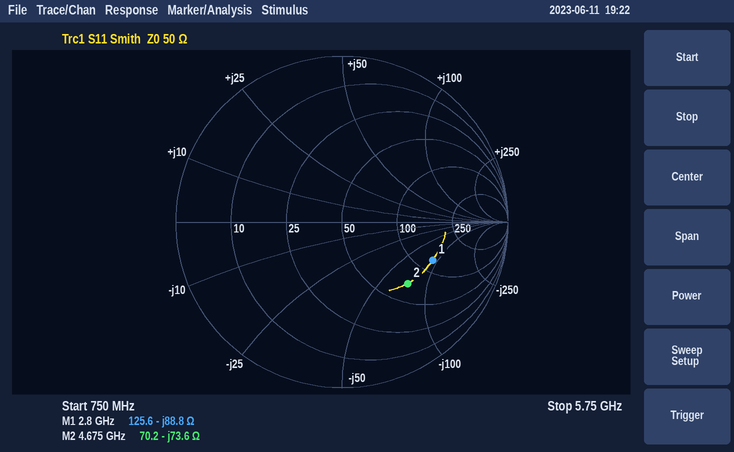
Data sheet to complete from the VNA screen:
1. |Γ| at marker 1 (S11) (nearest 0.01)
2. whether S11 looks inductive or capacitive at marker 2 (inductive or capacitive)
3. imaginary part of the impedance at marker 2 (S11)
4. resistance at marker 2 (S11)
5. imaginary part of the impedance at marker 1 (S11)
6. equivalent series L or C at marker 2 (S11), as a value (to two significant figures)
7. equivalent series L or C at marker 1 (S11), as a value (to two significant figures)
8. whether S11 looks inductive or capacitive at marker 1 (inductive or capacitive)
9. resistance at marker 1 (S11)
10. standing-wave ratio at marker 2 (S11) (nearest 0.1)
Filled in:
0.59
capacitive
-73.6 Ω
70.2 Ω
-88.8 Ω
460 fF
640 fF
capacitive
125.6 Ω
3.4
